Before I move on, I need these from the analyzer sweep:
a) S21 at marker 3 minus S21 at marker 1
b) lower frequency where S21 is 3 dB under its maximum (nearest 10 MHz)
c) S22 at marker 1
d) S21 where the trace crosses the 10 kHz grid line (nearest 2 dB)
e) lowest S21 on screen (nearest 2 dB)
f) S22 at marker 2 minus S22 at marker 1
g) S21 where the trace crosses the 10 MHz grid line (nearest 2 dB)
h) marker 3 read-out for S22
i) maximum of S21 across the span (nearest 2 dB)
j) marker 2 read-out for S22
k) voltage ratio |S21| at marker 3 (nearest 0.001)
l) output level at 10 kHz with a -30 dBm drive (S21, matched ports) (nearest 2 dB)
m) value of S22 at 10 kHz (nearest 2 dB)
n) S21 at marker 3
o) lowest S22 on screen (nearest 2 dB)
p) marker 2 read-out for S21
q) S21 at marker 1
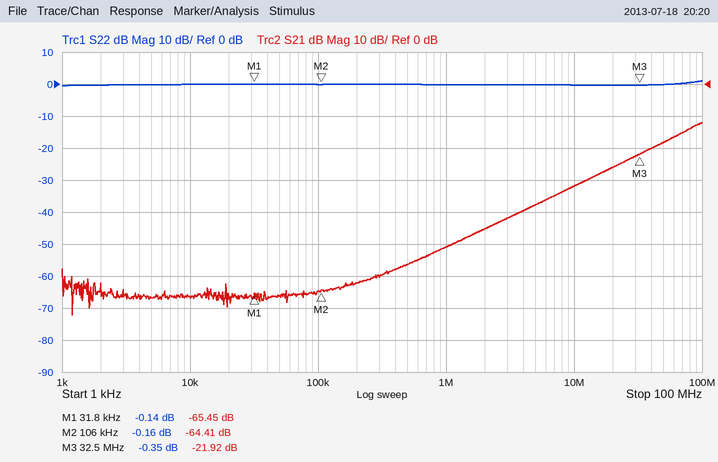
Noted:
43.53 dB
70 MHz
-0.14 dB
-66 dB
-72 dB
-0.02 dB
-32 dB
-0.35 dB
-12 dB
-0.16 dB
0.080
-96 dBm
0 dB
-21.92 dB
0 dB
-64.41 dB
-65.45 dB
